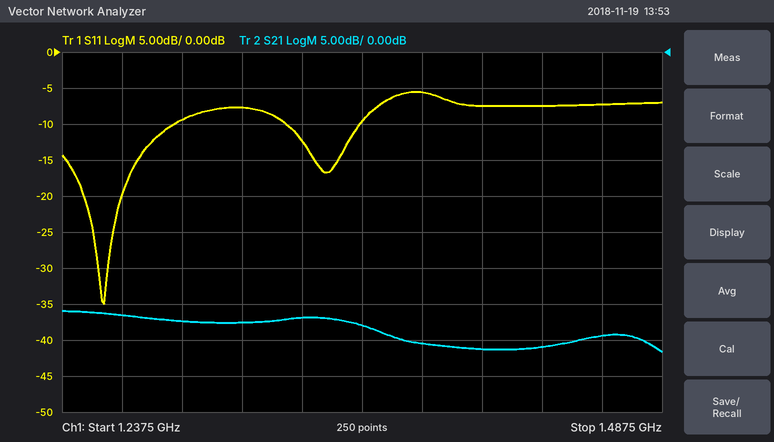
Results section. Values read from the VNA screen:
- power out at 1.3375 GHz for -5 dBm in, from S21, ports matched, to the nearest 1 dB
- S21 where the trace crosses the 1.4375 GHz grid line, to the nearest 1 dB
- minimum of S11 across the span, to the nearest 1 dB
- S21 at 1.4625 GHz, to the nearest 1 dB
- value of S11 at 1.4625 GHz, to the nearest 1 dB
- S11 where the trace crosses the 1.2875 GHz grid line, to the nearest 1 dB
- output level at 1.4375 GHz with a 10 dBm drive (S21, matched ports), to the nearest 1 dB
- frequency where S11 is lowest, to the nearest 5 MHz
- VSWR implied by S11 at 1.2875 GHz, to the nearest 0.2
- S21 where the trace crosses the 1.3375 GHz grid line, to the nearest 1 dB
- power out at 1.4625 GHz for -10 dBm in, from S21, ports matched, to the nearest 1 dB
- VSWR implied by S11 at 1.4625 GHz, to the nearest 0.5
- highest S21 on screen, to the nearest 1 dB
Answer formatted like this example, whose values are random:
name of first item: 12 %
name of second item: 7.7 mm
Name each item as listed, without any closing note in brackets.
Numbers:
power out at 1.3375 GHz for -5 dBm in, from S21, ports matched, to the nearest 1 dB: -42 dBm
S21 where the trace crosses the 1.4375 GHz grid line, to the nearest 1 dB: -41 dB
minimum of S11 across the span, to the nearest 1 dB: -35 dB
S21 at 1.4625 GHz, to the nearest 1 dB: -39 dB
value of S11 at 1.4625 GHz, to the nearest 1 dB: -7 dB
S11 where the trace crosses the 1.2875 GHz grid line, to the nearest 1 dB: -9 dB
output level at 1.4375 GHz with a 10 dBm drive (S21, matched ports), to the nearest 1 dB: -31 dBm
frequency where S11 is lowest, to the nearest 5 MHz: 1.255 GHz
VSWR implied by S11 at 1.2875 GHz, to the nearest 0.2: 2.0
S21 where the trace crosses the 1.3375 GHz grid line, to the nearest 1 dB: -37 dB
power out at 1.4625 GHz for -10 dBm in, from S21, ports matched, to the nearest 1 dB: -49 dBm
VSWR implied by S11 at 1.4625 GHz, to the nearest 0.5: 2.5
highest S21 on screen, to the nearest 1 dB: -36 dB
